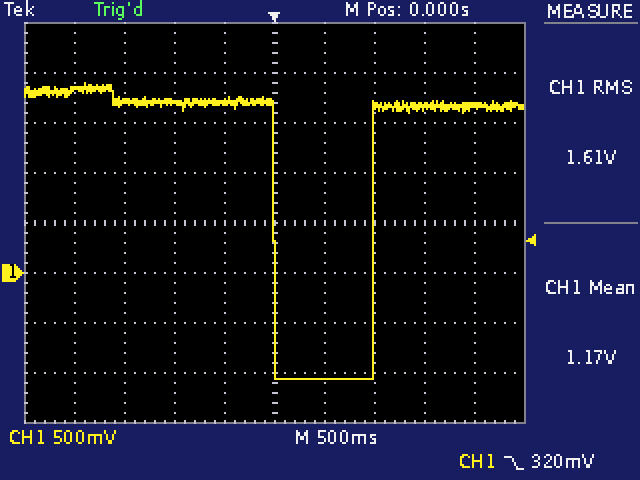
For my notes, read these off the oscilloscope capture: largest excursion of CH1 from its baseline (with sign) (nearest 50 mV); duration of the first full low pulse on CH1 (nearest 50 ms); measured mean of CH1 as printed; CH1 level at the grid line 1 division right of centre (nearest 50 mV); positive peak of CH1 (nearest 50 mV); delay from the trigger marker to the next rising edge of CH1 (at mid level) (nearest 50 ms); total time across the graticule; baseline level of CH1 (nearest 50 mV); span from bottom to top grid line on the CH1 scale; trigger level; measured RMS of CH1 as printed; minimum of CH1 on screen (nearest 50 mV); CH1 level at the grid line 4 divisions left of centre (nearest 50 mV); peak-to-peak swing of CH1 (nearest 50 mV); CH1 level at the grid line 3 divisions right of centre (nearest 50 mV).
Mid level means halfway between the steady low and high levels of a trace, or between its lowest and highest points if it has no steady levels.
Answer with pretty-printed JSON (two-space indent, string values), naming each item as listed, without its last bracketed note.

{
  "largest excursion of CH1 from its baseline (with sign)": "-2.75 V",
  "duration of the first full low pulse on CH1": "1.00 s",
  "measured mean of CH1 as printed": "1.17 V",
  "CH1 level at the grid line 1 division right of centre": "-1.05 V",
  "positive peak of CH1": "1.90 V",
  "delay from the trigger marker to the next rising edge of CH1 (at mid level)": "1.00 s",
  "total time across the graticule": "5 s",
  "baseline level of CH1": "1.70 V",
  "span from bottom to top grid line on the CH1 scale": "4 V",
  "trigger level": "320 mV",
  "measured RMS of CH1 as printed": "1.61 V",
  "minimum of CH1 on screen": "-1.05 V",
  "CH1 level at the grid line 4 divisions left of centre": "1.85 V",
  "peak-to-peak swing of CH1": "2.95 V",
  "CH1 level at the grid line 3 divisions right of centre": "1.65 V"
}
